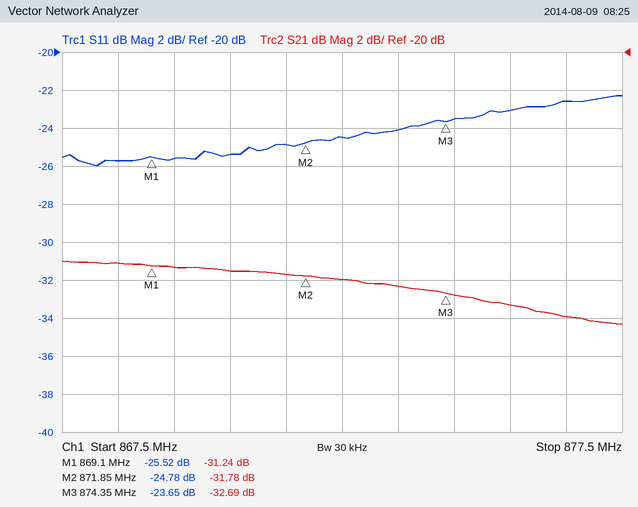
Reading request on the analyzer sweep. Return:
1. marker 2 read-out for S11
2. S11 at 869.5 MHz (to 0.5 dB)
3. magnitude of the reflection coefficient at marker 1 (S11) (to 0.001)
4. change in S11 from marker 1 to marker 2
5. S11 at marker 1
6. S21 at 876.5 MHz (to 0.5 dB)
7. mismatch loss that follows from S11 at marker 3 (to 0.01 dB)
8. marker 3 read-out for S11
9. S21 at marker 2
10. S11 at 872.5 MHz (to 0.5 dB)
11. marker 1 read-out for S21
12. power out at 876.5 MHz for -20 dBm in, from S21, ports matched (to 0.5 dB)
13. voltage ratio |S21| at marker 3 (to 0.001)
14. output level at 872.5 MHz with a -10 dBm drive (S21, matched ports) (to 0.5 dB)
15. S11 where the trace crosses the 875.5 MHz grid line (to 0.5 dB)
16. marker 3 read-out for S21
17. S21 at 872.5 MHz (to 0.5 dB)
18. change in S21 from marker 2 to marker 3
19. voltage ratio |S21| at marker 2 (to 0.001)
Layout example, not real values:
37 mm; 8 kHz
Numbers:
-24.78 dB; -25.5 dB; 0.053; 0.74 dB; -25.52 dB; -34.0 dB; 0.02 dB; -23.65 dB; -31.78 dB; -24.5 dB; -31.24 dB; -54.0 dBm; 0.023; -42.0 dBm; -23.0 dB; -32.69 dB; -32.0 dB; -0.91 dB; 0.026
